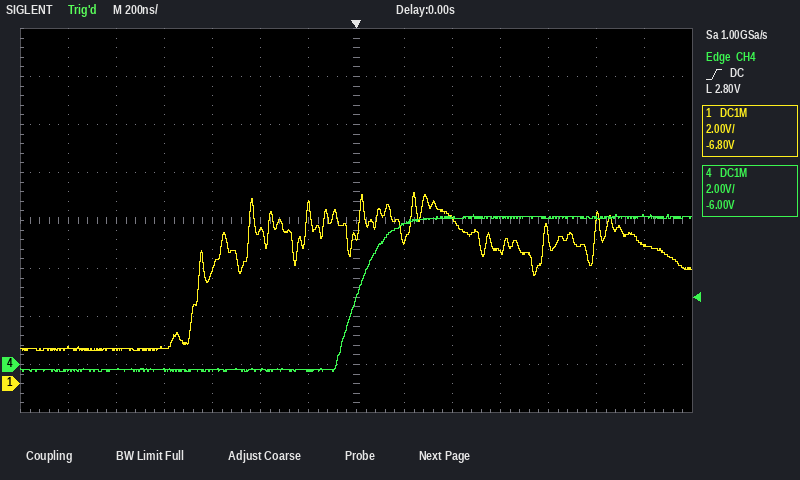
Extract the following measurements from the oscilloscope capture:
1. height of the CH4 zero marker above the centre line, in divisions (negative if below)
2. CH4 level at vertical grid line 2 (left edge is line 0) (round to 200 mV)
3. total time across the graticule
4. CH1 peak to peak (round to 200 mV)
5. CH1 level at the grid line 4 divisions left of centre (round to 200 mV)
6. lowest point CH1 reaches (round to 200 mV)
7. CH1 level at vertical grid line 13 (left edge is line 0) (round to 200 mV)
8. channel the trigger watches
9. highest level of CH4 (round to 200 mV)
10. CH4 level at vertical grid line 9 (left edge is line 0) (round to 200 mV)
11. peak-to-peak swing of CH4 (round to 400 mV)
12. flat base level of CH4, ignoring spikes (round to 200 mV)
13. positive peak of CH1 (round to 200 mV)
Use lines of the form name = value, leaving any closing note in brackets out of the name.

height of the CH4 zero marker above the centre line, in divisions = -3.0 div
CH4 level at vertical grid line 2 (left edge is line 0) = -200 mV
total time across the graticule = 2.8 µs
CH1 peak to peak = 6.6 V
CH1 level at the grid line 4 divisions left of centre = 1.4 V
lowest point CH1 reaches = 1.4 V
CH1 level at vertical grid line 13 (left edge is line 0) = 5.8 V
channel the trigger watches = CH4
highest level of CH4 = 6.2 V
CH4 level at vertical grid line 9 (left edge is line 0) = 6.2 V
peak-to-peak swing of CH4 = 6.4 V
flat base level of CH4, ignoring spikes = -200 mV
positive peak of CH1 = 8.0 V
